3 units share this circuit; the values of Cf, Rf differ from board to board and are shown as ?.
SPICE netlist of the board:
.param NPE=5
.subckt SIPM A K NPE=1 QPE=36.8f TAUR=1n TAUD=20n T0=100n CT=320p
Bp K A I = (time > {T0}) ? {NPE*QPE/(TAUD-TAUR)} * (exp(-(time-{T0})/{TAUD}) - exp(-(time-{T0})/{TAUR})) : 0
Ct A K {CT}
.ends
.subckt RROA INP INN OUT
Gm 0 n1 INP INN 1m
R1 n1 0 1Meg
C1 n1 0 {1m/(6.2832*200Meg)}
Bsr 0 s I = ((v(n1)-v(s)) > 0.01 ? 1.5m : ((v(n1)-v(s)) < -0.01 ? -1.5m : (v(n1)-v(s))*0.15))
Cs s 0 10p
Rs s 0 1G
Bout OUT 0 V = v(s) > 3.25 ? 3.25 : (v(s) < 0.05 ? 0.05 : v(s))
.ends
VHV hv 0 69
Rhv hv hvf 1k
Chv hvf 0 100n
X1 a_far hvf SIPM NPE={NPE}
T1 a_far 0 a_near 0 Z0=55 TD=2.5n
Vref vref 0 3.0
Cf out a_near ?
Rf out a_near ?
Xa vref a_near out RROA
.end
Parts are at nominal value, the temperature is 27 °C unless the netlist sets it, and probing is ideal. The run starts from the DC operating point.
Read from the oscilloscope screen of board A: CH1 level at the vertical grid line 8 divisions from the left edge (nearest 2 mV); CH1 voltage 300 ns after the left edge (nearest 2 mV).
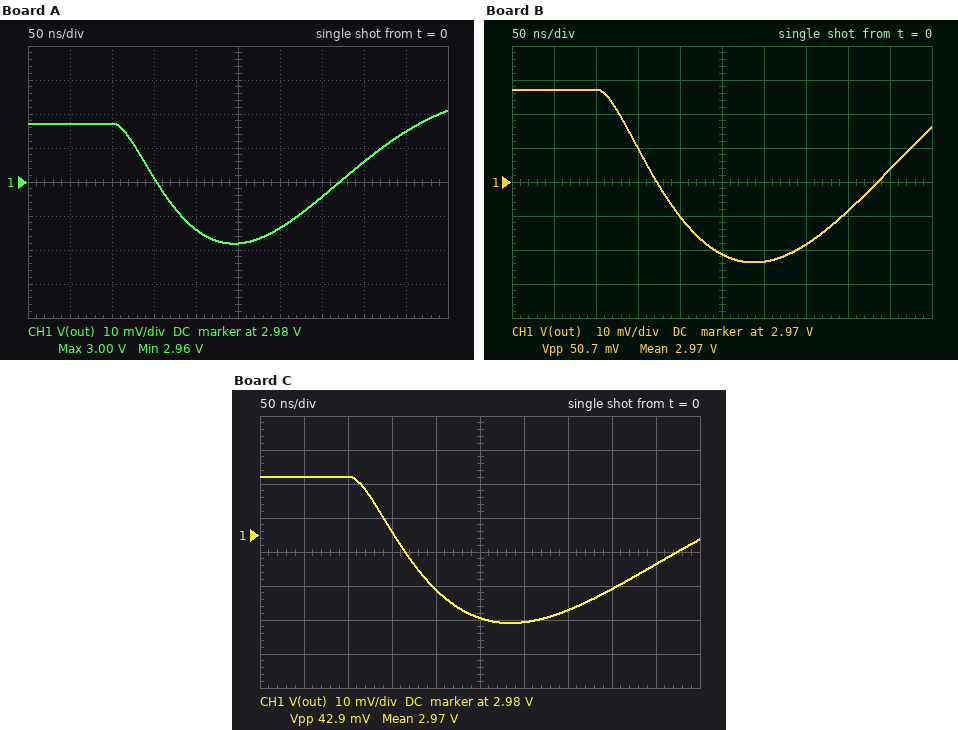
2.986 V
2.966 V
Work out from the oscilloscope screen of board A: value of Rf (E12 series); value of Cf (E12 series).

33 kΩ
2.2 pF
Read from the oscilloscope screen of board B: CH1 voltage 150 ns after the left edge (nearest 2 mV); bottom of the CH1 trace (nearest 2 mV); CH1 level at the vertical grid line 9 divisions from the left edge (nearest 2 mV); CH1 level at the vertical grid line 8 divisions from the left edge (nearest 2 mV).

2.980 V
2.946 V
2.974 V
2.962 V
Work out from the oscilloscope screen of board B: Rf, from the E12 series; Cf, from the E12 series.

56 kΩ
1.2 pF
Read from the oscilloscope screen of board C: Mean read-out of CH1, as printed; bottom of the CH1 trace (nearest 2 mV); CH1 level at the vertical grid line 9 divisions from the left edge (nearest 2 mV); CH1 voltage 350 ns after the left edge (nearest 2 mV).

2.97 V
2.954 V
2.972 V
2.958 V
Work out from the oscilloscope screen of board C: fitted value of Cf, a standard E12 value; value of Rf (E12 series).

2.2 pF
68 kΩ
